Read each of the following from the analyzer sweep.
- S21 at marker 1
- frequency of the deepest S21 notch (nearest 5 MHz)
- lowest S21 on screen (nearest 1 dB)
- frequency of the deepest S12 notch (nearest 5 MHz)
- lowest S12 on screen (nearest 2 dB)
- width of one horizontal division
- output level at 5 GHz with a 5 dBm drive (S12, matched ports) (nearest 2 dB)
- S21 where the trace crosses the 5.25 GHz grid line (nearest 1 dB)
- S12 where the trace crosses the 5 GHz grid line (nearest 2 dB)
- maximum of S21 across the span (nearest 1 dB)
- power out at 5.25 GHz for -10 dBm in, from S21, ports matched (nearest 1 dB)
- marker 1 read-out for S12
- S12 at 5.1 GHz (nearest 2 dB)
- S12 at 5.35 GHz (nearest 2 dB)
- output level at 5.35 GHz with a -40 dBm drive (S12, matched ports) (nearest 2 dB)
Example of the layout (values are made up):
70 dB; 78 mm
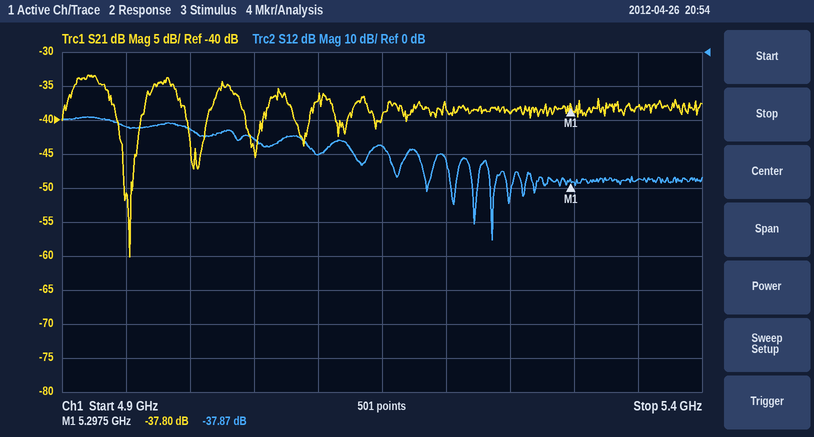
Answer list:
-37.80 dB; 4.955 GHz; -60 dB; 5.235 GHz; -56 dB; 50 MHz; -18 dBm; -39 dB; -22 dB; -33 dB; -49 dBm; -37.87 dB; -30 dB; -38 dB; -78 dBm
